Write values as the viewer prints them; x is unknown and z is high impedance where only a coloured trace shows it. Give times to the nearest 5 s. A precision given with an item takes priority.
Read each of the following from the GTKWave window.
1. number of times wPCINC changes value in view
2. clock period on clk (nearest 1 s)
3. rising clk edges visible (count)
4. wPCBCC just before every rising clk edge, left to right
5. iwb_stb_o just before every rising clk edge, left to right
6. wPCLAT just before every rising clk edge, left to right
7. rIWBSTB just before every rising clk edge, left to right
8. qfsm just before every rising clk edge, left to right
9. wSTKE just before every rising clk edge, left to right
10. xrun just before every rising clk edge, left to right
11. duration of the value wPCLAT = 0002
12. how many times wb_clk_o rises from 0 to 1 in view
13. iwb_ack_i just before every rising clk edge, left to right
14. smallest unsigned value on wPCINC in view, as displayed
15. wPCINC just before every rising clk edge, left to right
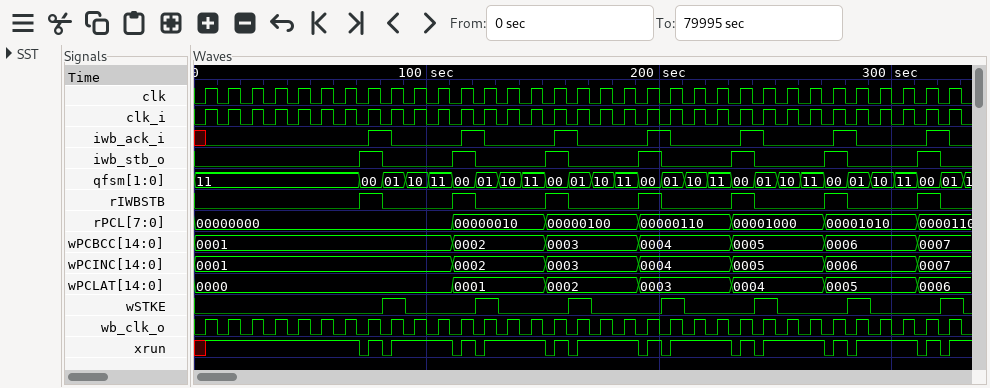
6
10 s
33
0001, 0001, 0001, 0001, 0001, 0001, 0001, 0001, 0001, 0001, 0001, 0002, 0002, 0002, 0002, 0003, 0003, 0003, 0003, 0004, 0004, 0004, 0004, 0005, 0005, 0005, 0005, 0006, 0006, 0006, 0006, 0007, 0007
0 0 0 0 0 0 0 1 0 0 0 1 0 0 0 1 0 0 0 1 0 0 0 1 0 0 0 1 0 0 0 1 0
0000, 0000, 0000, 0000, 0000, 0000, 0000, 0000, 0000, 0000, 0000, 0001, 0001, 0001, 0001, 0002, 0002, 0002, 0002, 0003, 0003, 0003, 0003, 0004, 0004, 0004, 0004, 0005, 0005, 0005, 0005, 0006, 0006
0 0 0 0 0 0 0 1 0 0 0 1 0 0 0 1 0 0 0 1 0 0 0 1 0 0 0 1 0 0 0 1 0
11, 11, 11, 11, 11, 11, 11, 00, 01, 10, 11, 00, 01, 10, 11, 00, 01, 10, 11, 00, 01, 10, 11, 00, 01, 10, 11, 00, 01, 10, 11, 00, 01
0 0 0 0 0 0 0 0 1 0 0 0 1 0 0 0 1 0 0 0 1 0 0 0 1 0 0 0 1 0 0 0 1
x 1 1 1 1 1 1 0 0 1 1 0 0 1 1 0 0 1 1 0 0 1 1 0 0 1 1 0 0 1 1 0 0
40 s
33
x 0 0 0 0 0 0 0 1 0 0 0 1 0 0 0 1 0 0 0 1 0 0 0 1 0 0 0 1 0 0 0 1
0001
0001, 0001, 0001, 0001, 0001, 0001, 0001, 0001, 0001, 0001, 0001, 0002, 0002, 0002, 0002, 0003, 0003, 0003, 0003, 0004, 0004, 0004, 0004, 0005, 0005, 0005, 0005, 0006, 0006, 0006, 0006, 0007, 0007
